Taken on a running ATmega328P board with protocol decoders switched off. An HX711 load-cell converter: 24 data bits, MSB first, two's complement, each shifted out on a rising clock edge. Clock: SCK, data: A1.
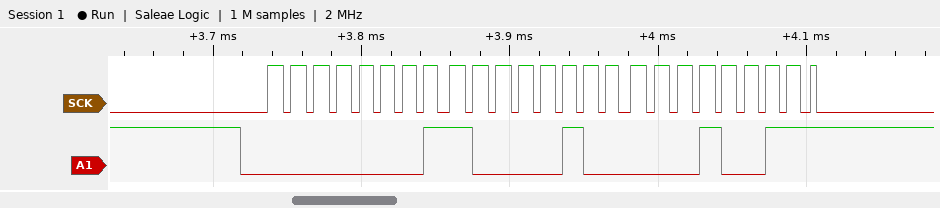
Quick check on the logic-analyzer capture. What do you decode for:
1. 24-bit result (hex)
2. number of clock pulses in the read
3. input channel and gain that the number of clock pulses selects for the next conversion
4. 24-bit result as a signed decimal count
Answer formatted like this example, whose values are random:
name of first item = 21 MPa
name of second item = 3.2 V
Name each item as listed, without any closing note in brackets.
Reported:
24-bit result = 0x018413
number of clock pulses in the read = 25
input channel and gain that the number of clock pulses selects for the next conversion = channel A, gain 128
24-bit result as a signed decimal count = 99347
